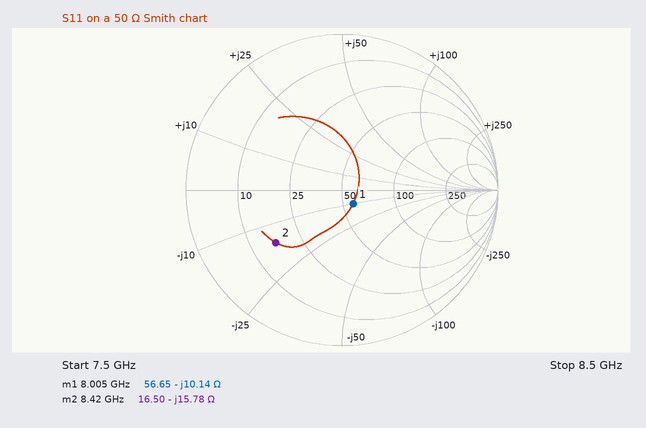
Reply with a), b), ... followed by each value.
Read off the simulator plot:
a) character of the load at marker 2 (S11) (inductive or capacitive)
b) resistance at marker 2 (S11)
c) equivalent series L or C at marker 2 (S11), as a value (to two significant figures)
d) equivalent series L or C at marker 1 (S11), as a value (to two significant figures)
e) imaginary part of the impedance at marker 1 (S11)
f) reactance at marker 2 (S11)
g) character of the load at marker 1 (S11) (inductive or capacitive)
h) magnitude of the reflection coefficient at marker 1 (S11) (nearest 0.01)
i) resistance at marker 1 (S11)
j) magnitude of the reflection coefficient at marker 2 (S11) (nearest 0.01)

a) capacitive
b) 16.50 Ω
c) 1.2 pF
d) 2.0 pF
e) -10.14 Ω
f) -15.78 Ω
g) capacitive
h) 0.11
i) 56.65 Ω
j) 0.54
